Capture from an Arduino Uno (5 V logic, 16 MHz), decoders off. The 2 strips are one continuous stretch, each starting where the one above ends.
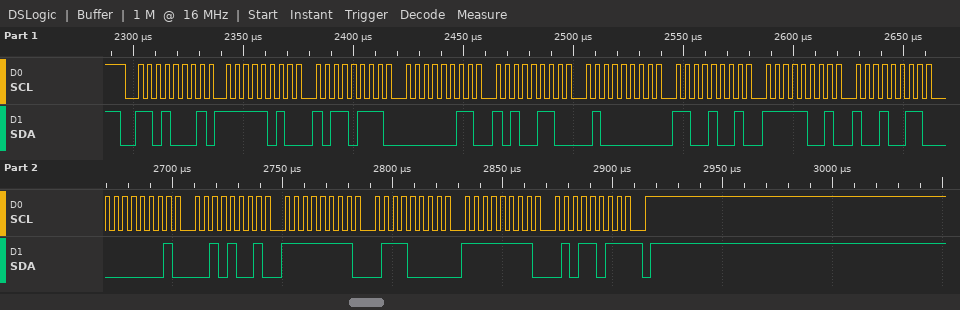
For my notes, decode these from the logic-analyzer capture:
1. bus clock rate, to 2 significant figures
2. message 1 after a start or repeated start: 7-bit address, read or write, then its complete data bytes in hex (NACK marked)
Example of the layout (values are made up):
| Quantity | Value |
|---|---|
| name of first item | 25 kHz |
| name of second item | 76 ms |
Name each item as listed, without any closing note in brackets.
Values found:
| Quantity | Value |
|---|---|
| bus clock rate, to 2 significant figures | 250 kHz |
| message 1 after a start or repeated start: 7-bit address, read or write, then its complete data bytes in hex | 0x68 read: FA B7 03 A6 40 C9 F9 93 01 29 FF 70 FF 5B NACK |
